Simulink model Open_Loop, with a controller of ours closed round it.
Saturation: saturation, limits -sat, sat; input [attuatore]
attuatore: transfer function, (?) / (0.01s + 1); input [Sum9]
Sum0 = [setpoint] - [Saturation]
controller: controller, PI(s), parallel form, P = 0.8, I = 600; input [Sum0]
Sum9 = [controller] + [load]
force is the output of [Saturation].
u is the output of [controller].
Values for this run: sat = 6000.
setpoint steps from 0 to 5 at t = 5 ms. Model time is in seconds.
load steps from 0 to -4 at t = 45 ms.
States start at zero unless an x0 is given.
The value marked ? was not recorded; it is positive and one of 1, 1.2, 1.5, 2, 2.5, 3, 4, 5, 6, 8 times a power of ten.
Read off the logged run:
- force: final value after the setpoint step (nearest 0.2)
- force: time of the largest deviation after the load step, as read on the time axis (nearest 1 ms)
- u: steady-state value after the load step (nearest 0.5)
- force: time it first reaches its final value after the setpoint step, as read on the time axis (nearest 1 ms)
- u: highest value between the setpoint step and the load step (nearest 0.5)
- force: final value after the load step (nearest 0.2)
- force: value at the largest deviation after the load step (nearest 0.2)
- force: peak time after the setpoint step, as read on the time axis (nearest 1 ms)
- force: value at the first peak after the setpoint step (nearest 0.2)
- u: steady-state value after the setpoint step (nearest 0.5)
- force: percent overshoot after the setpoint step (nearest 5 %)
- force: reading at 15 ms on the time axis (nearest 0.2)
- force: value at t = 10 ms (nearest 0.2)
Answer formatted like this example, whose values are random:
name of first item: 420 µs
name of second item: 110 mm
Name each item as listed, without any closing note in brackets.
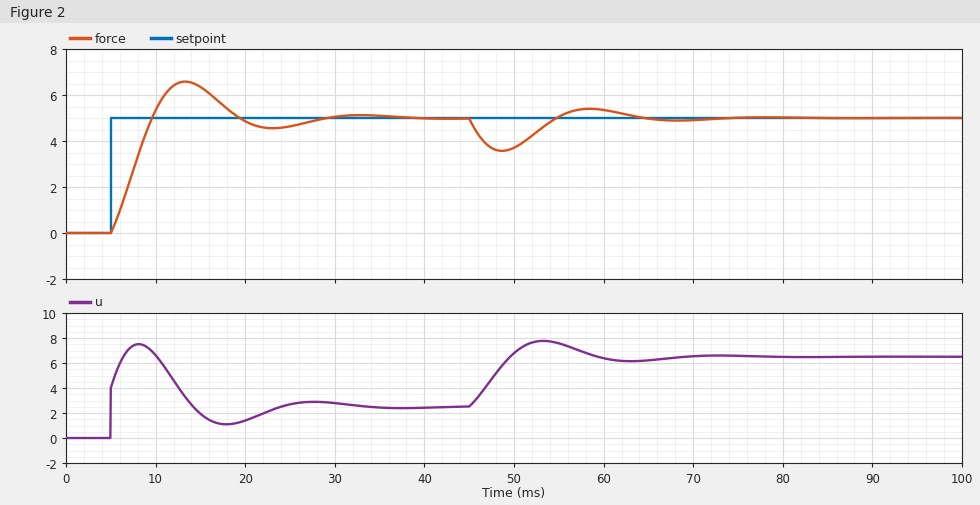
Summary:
force: final value after the setpoint step: 5.0
force: time of the largest deviation after the load step, as read on the time axis: 49 ms
u: steady-state value after the load step: 6.5
force: time it first reaches its final value after the setpoint step, as read on the time axis: 10 ms
u: highest value between the setpoint step and the load step: 7.5
force: final value after the load step: 5.0
force: value at the largest deviation after the load step: 3.6
force: peak time after the setpoint step, as read on the time axis: 13 ms
force: value at the first peak after the setpoint step: 6.6
u: steady-state value after the setpoint step: 2.5
force: percent overshoot after the setpoint step: 30 %
force: reading at 15 ms on the time axis: 6.4
force: value at t = 10 ms: 5.4
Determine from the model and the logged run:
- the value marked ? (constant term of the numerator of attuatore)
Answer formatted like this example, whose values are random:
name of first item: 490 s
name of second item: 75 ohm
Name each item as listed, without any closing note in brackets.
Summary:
the value marked ?: 2
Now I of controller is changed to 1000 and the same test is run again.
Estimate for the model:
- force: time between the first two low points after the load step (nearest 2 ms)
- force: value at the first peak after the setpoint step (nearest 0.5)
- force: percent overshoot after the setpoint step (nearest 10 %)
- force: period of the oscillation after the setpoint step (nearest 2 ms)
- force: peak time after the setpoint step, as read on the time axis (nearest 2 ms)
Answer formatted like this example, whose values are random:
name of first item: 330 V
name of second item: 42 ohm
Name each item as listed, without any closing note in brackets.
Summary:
force: time between the first two low points after the load step: 14 ms
force: value at the first peak after the setpoint step: 7.0
force: percent overshoot after the setpoint step: 40 %
force: period of the oscillation after the setpoint step: 14 ms
force: peak time after the setpoint step, as read on the time axis: 12 ms
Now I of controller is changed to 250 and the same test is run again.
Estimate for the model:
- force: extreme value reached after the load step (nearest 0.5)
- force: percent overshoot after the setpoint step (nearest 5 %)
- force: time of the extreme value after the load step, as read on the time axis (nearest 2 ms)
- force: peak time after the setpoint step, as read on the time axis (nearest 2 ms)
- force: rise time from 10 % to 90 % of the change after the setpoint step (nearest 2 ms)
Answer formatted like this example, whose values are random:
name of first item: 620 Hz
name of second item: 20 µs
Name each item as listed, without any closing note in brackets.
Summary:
force: extreme value reached after the load step: 3.0
force: percent overshoot after the setpoint step: 15 %
force: time of the extreme value after the load step, as read on the time axis: 50 ms
force: peak time after the setpoint step, as read on the time axis: 18 ms
force: rise time from 10 % to 90 % of the change after the setpoint step: 6 ms
